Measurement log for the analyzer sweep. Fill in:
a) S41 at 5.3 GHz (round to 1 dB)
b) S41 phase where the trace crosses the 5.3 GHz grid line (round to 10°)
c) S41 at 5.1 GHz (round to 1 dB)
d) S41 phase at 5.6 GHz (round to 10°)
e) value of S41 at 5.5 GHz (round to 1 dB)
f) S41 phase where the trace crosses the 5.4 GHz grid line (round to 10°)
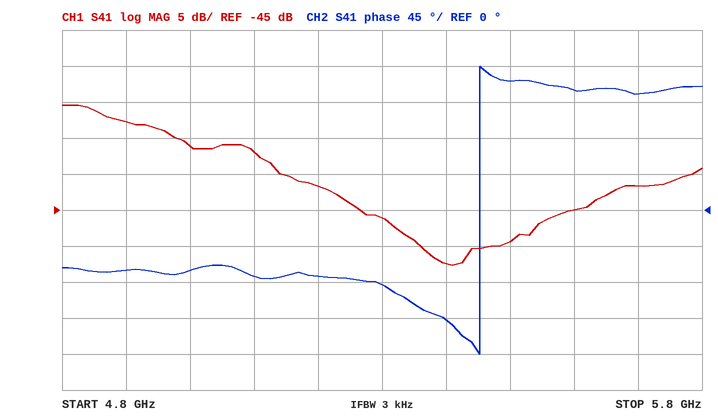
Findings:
-46 dB
-90°
-37 dB
150°
-49 dB
-140°
